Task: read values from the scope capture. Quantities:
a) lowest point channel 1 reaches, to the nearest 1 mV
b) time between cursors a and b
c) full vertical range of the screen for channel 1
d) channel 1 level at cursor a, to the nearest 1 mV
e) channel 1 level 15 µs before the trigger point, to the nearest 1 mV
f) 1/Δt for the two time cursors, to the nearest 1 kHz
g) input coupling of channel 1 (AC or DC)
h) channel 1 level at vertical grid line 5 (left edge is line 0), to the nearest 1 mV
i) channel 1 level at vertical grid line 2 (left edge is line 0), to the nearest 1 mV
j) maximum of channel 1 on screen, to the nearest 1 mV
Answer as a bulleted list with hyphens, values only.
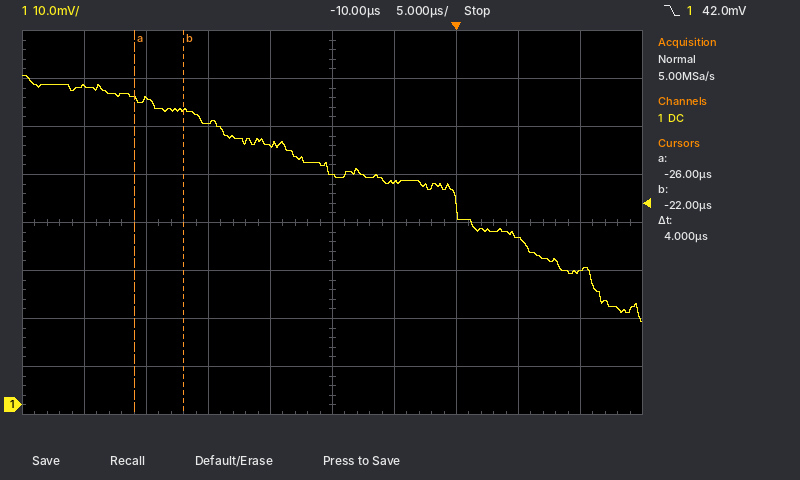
- 17 mV
- 4 µs
- 80 mV
- 64 mV
- 54 mV
- 250 kHz
- DC
- 48 mV
- 64 mV
- 69 mV
